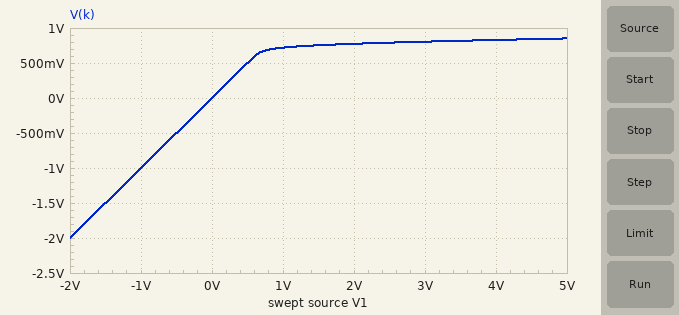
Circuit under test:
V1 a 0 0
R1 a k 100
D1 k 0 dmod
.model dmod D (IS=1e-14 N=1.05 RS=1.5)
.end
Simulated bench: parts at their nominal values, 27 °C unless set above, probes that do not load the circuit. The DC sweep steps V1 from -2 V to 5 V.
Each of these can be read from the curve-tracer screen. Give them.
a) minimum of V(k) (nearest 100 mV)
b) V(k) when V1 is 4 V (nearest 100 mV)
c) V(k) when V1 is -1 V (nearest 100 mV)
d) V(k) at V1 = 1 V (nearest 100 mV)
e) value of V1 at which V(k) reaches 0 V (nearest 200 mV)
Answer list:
-2.0 V
800 mV
-1.0 V
700 mV
0 V
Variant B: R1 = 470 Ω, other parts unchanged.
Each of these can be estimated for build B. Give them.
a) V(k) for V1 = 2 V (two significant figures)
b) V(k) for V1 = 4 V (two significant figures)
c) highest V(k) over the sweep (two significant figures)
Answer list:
720 mV
750 mV
760 mV
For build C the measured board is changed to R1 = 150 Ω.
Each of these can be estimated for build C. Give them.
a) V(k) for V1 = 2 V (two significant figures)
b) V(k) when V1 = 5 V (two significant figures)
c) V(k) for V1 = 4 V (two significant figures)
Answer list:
760 mV
820 mV
800 mV
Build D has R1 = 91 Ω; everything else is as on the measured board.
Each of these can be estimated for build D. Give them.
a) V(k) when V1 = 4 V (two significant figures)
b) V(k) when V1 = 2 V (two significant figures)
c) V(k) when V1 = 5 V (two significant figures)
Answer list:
840 mV
780 mV
860 mV
